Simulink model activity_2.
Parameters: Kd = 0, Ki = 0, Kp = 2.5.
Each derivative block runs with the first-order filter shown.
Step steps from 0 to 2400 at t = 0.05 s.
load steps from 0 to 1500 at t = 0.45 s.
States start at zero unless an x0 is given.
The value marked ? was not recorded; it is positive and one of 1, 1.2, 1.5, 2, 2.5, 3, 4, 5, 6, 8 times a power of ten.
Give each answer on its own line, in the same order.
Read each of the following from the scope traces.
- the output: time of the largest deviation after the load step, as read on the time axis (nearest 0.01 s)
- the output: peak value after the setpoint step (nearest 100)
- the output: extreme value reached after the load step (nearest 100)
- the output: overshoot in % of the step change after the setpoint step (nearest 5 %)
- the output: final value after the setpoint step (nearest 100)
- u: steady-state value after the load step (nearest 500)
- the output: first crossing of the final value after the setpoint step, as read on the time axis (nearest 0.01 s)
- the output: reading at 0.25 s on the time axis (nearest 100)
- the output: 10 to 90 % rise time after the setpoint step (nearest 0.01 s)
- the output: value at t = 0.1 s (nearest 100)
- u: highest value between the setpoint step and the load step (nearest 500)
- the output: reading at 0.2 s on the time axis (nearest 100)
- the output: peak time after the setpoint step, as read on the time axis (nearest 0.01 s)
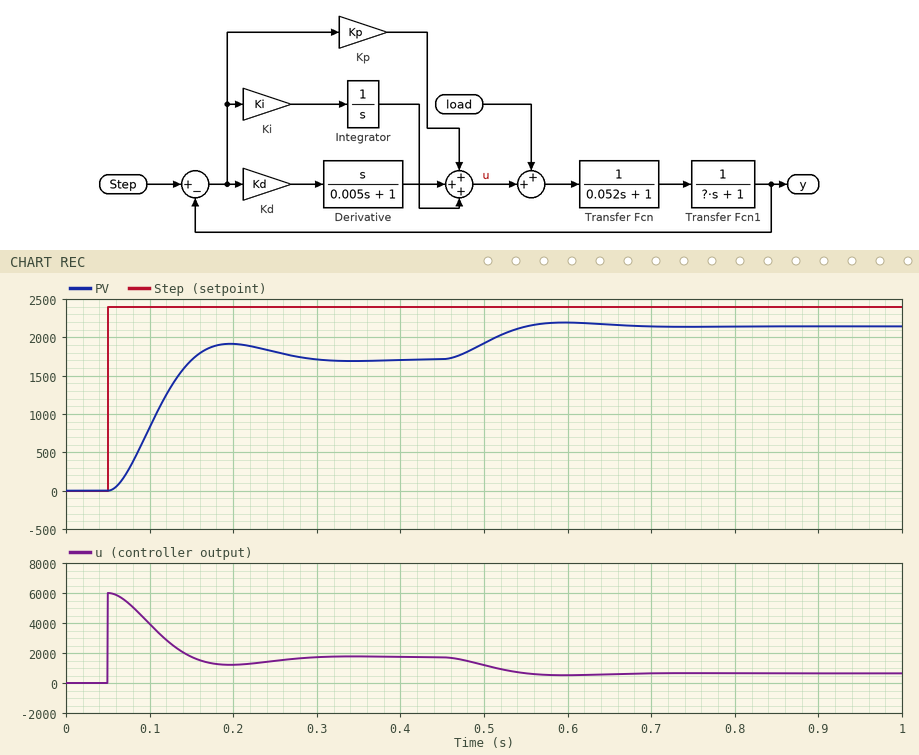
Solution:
0.60 s
1900
2200
10 %
1700
500
0.15 s
1800
0.07 s
800
6000
1900
0.20 s
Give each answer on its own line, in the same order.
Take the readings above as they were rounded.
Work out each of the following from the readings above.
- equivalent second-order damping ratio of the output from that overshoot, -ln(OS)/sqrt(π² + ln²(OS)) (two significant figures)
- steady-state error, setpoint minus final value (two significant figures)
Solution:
0.59
700
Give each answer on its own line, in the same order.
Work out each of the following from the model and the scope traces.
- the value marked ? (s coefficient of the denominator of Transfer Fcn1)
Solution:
0.1
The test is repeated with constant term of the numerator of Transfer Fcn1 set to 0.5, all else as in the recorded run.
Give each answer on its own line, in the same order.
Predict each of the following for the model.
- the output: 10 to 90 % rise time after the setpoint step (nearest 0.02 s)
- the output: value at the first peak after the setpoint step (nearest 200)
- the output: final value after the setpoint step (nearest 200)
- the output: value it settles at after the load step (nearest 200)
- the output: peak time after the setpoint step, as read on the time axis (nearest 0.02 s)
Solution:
0.10 s
1400
1400
1600
0.26 s
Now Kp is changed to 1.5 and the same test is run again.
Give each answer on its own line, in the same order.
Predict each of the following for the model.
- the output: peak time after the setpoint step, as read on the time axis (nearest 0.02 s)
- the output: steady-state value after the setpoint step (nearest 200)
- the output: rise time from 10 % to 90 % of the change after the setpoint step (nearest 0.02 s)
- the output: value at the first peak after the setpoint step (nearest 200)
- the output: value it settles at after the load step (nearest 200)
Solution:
0.24 s
1400
0.10 s
1600
2000
